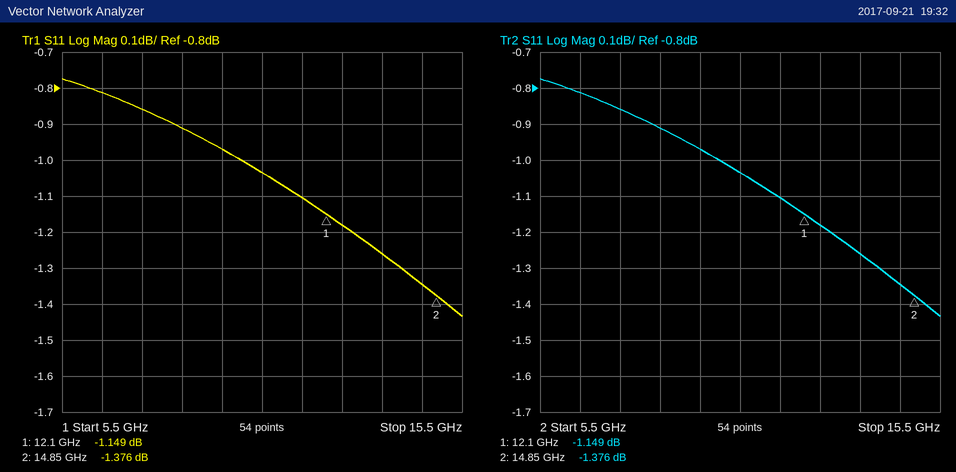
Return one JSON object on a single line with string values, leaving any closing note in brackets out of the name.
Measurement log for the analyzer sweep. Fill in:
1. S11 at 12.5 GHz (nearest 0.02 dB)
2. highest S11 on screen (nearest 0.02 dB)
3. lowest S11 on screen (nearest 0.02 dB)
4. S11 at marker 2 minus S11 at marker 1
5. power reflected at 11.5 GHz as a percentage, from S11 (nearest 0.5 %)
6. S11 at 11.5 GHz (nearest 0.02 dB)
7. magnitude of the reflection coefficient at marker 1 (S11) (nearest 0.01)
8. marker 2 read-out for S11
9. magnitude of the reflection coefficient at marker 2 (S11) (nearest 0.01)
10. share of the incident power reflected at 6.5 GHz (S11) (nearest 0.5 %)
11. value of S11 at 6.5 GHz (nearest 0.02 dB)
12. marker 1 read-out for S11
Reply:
{"S11 at 12.5 GHz": "-1.18 dB", "highest S11 on screen": "-0.78 dB", "lowest S11 on screen": "-1.44 dB", "S11 at marker 2 minus S11 at marker 1": "-0.227 dB", "power reflected at 11.5 GHz as a percentage, from S11": "77.5 %", "S11 at 11.5 GHz": "-1.10 dB", "magnitude of the reflection coefficient at marker 1 (S11)": "0.88", "marker 2 read-out for S11": "-1.376 dB", "magnitude of the reflection coefficient at marker 2 (S11)": "0.85", "share of the incident power reflected at 6.5 GHz (S11)": "83.0 %", "value of S11 at 6.5 GHz": "-0.82 dB", "marker 1 read-out for S11": "-1.149 dB"}
